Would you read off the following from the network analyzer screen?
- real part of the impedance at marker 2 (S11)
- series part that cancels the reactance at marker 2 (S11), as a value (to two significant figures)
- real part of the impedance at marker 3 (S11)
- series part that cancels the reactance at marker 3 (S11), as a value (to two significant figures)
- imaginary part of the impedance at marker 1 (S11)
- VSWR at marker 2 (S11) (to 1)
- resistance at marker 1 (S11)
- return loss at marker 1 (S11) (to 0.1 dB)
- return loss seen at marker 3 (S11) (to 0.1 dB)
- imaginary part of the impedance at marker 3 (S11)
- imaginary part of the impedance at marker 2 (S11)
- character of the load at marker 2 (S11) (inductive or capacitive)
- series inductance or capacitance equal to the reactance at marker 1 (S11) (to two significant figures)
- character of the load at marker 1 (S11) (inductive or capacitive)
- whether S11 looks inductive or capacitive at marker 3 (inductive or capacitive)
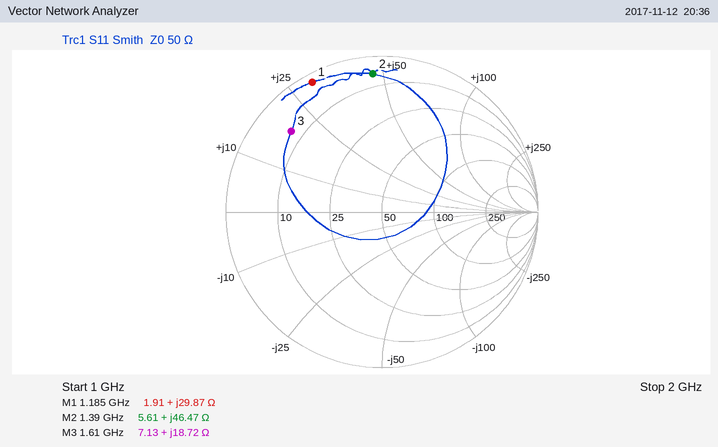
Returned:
5.61 Ω
2.5 pF
7.13 Ω
5.3 pF
+29.87 Ω
17
1.91 Ω
0.5 dB
2.2 dB
+18.72 Ω
+46.47 Ω
inductive
4.0 nH
inductive
inductive
